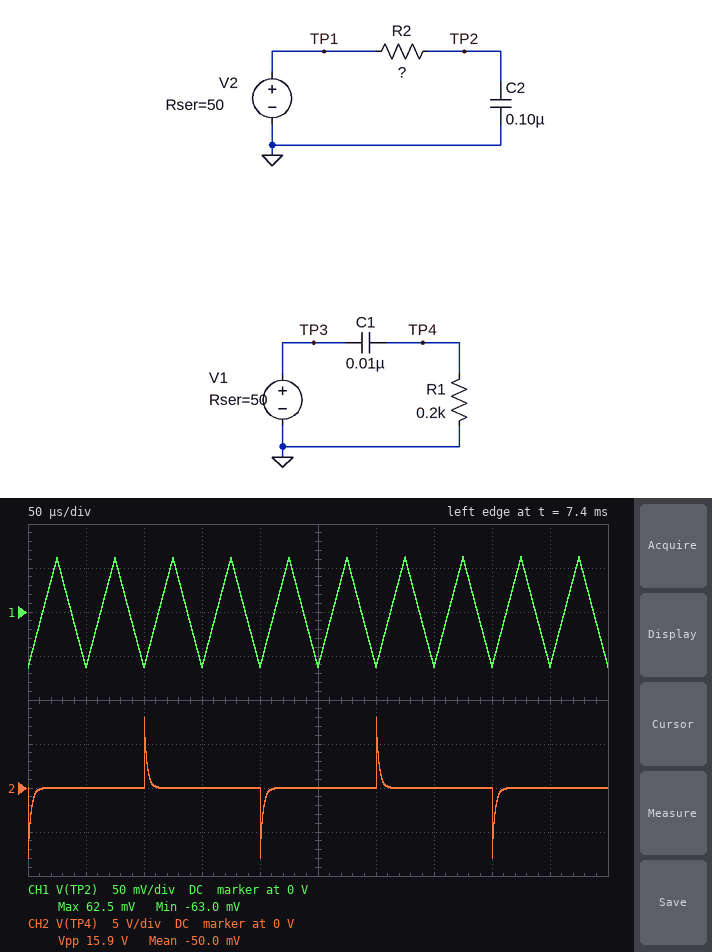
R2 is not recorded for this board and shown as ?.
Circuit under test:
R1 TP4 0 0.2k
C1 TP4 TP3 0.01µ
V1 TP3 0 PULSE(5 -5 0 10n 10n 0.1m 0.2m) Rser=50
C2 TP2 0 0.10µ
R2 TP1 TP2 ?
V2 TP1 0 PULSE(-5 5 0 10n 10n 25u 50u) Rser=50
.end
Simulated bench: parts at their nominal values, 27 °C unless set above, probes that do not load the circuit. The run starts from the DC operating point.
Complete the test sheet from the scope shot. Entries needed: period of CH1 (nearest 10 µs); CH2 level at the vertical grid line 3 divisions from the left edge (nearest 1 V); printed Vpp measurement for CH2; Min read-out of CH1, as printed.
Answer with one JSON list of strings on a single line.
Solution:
["50 µs", "0 V", "15.9 V", "-63.0 mV"]
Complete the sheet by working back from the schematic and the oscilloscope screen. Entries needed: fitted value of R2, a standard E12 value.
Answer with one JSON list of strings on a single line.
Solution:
["10 kΩ"]
